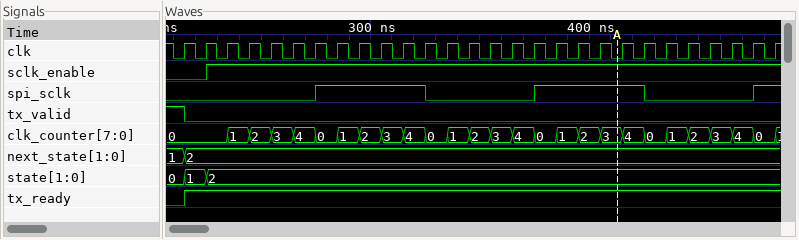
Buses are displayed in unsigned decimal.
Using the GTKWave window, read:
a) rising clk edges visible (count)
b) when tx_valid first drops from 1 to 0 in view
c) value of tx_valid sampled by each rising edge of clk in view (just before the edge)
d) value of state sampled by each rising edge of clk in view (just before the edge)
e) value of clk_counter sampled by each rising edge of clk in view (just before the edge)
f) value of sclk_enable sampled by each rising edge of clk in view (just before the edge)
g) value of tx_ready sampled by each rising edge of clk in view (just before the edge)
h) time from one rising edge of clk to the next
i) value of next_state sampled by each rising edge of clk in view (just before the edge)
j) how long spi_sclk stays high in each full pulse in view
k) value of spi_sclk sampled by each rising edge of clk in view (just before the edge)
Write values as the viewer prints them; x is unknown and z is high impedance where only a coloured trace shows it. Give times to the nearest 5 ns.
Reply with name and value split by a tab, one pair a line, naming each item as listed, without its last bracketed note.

rising clk edges visible	28
when tx_valid first drops from 1 to 0 in view	215 ns
value of tx_valid sampled by each rising edge of clk in view	1 0 0 0 0 0 0 0 0 0 0 0 0 0 0 0 0 0 0 0 0 0 0 0 0 0 0 0
value of state sampled by each rising edge of clk in view	0, 1, 2, 2, 2, 2, 2, 2, 2, 2, 2, 2, 2, 2, 2, 2, 2, 2, 2, 2, 2, 2, 2, 2, 2, 2, 2, 2
value of clk_counter sampled by each rising edge of clk in view	0, 0, 0, 1, 2, 3, 4, 0, 1, 2, 3, 4, 0, 1, 2, 3, 4, 0, 1, 2, 3, 4, 0, 1, 2, 3, 4, 0
value of sclk_enable sampled by each rising edge of clk in view	0 0 1 1 1 1 1 1 1 1 1 1 1 1 1 1 1 1 1 1 1 1 1 1 1 1 1 1
value of tx_ready sampled by each rising edge of clk in view	0 1 1 1 1 1 1 1 1 1 1 1 1 1 1 1 1 1 1 1 1 1 1 1 1 1 1 1
time from one rising edge of clk to the next	10 ns
value of next_state sampled by each rising edge of clk in view	1, 2, 2, 2, 2, 2, 2, 2, 2, 2, 2, 2, 2, 2, 2, 2, 2, 2, 2, 2, 2, 2, 2, 2, 2, 2, 2, 2
how long spi_sclk stays high in each full pulse in view	50 ns, 50 ns
value of spi_sclk sampled by each rising edge of clk in view	0 0 0 0 0 0 0 1 1 1 1 1 0 0 0 0 0 1 1 1 1 1 0 0 0 0 0 1
